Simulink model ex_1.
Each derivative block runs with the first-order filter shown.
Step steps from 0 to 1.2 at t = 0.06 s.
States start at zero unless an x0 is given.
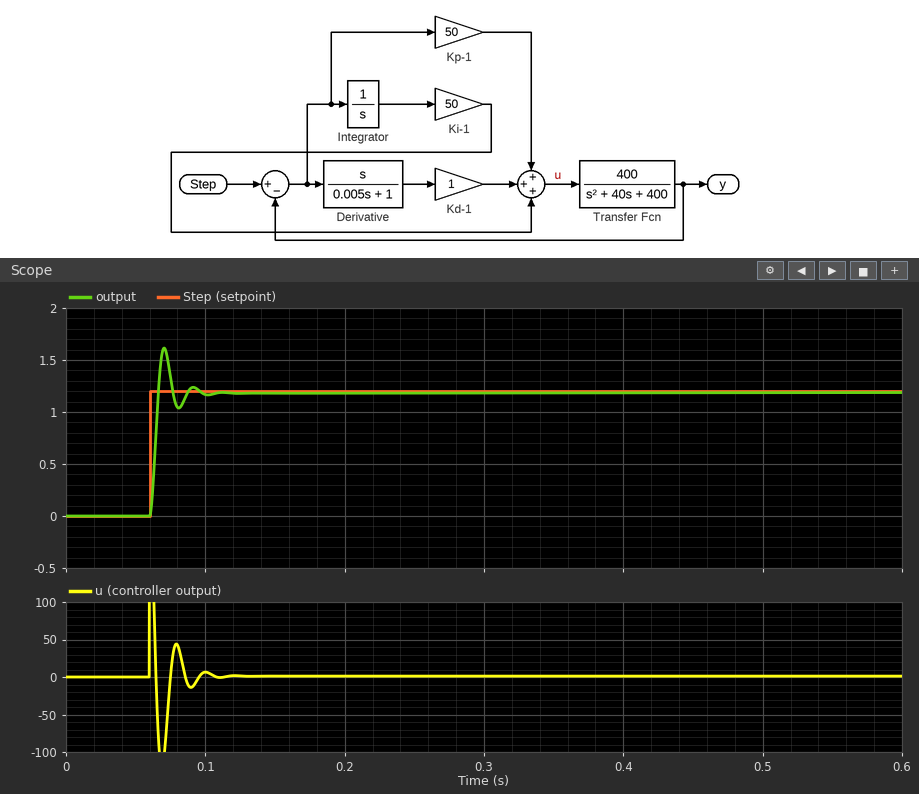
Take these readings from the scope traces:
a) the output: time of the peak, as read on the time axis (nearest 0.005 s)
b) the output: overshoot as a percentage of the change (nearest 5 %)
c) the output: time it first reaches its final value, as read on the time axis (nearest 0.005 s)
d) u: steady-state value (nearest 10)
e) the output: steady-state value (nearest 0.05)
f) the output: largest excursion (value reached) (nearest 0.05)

0.070 s
35 %
0.065 s
0
1.20
1.60
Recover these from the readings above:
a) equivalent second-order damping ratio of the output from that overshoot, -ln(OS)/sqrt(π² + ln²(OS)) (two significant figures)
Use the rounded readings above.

0.32
